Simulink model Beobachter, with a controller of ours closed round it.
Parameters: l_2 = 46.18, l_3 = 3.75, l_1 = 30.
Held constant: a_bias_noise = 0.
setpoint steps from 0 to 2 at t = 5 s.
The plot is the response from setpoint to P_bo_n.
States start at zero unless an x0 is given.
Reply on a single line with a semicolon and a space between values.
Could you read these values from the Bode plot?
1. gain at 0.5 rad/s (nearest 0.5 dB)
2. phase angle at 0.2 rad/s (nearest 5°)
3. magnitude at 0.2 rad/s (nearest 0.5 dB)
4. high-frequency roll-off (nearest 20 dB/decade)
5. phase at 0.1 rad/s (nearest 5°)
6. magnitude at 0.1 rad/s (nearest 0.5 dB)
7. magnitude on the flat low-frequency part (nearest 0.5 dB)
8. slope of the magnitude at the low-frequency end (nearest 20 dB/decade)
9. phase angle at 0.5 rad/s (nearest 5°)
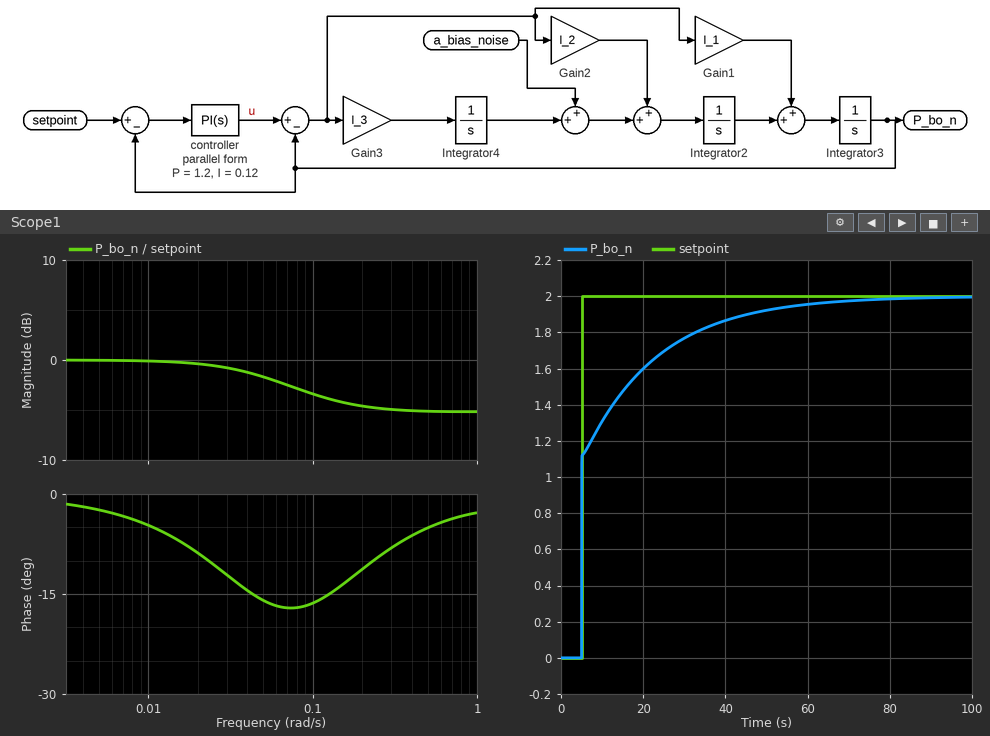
-5.0 dB; -10°; -4.5 dB; 0 dB/decade; -15°; -3.5 dB; 0.0 dB; 0 dB/decade; -5°
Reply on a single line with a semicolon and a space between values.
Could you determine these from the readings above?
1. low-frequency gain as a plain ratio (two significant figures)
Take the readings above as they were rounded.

1.0
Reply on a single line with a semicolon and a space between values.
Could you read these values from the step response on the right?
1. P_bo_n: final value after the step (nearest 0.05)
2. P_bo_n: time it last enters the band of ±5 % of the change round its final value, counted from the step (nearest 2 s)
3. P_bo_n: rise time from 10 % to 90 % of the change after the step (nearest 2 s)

2.00; 40 s; 28 s
